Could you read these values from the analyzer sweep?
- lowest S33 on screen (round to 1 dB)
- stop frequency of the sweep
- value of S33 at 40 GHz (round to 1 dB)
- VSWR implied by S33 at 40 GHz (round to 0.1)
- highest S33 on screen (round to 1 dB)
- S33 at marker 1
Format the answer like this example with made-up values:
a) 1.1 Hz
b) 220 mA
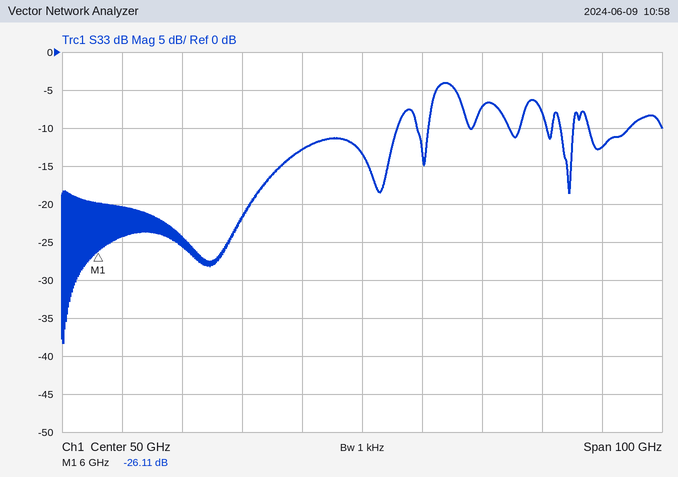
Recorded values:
a) -38 dB
b) 100 GHz
c) -13 dB
d) 1.6
e) -4 dB
f) -26.11 dB
